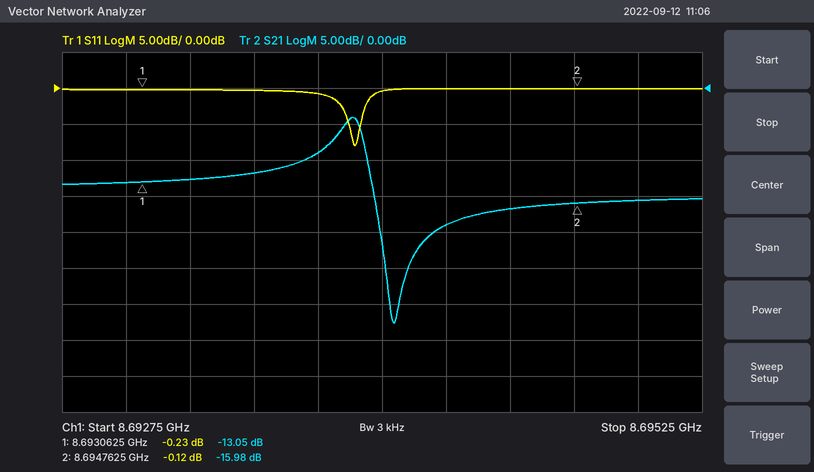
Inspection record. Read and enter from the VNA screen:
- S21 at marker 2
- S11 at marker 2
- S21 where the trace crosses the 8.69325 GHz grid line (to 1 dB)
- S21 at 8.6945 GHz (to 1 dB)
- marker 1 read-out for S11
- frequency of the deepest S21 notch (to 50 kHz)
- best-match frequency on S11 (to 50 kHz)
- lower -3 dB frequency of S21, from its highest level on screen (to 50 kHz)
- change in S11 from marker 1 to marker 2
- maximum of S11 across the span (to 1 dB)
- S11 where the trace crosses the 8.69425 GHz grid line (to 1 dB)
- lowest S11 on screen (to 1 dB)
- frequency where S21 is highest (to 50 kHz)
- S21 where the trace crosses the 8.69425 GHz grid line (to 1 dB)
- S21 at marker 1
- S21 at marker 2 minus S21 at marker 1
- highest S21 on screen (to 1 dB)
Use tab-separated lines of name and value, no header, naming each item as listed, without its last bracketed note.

S21 at marker 2	-15.98 dB
S11 at marker 2	-0.12 dB
S21 where the trace crosses the 8.69325 GHz grid line	-13 dB
S21 at 8.6945 GHz	-17 dB
marker 1 read-out for S11	-0.23 dB
frequency of the deepest S21 notch	8.69405 GHz
best-match frequency on S11	8.69390 GHz
lower -3 dB frequency of S21, from its highest level on screen	8.69380 GHz
change in S11 from marker 1 to marker 2	0.11 dB
maximum of S11 across the span	0 dB
S11 where the trace crosses the 8.69425 GHz grid line	0 dB
lowest S11 on screen	-8 dB
frequency where S21 is highest	8.69390 GHz
S21 where the trace crosses the 8.69425 GHz grid line	-19 dB
S21 at marker 1	-13.05 dB
S21 at marker 2 minus S21 at marker 1	-2.93 dB
highest S21 on screen	-4 dB
